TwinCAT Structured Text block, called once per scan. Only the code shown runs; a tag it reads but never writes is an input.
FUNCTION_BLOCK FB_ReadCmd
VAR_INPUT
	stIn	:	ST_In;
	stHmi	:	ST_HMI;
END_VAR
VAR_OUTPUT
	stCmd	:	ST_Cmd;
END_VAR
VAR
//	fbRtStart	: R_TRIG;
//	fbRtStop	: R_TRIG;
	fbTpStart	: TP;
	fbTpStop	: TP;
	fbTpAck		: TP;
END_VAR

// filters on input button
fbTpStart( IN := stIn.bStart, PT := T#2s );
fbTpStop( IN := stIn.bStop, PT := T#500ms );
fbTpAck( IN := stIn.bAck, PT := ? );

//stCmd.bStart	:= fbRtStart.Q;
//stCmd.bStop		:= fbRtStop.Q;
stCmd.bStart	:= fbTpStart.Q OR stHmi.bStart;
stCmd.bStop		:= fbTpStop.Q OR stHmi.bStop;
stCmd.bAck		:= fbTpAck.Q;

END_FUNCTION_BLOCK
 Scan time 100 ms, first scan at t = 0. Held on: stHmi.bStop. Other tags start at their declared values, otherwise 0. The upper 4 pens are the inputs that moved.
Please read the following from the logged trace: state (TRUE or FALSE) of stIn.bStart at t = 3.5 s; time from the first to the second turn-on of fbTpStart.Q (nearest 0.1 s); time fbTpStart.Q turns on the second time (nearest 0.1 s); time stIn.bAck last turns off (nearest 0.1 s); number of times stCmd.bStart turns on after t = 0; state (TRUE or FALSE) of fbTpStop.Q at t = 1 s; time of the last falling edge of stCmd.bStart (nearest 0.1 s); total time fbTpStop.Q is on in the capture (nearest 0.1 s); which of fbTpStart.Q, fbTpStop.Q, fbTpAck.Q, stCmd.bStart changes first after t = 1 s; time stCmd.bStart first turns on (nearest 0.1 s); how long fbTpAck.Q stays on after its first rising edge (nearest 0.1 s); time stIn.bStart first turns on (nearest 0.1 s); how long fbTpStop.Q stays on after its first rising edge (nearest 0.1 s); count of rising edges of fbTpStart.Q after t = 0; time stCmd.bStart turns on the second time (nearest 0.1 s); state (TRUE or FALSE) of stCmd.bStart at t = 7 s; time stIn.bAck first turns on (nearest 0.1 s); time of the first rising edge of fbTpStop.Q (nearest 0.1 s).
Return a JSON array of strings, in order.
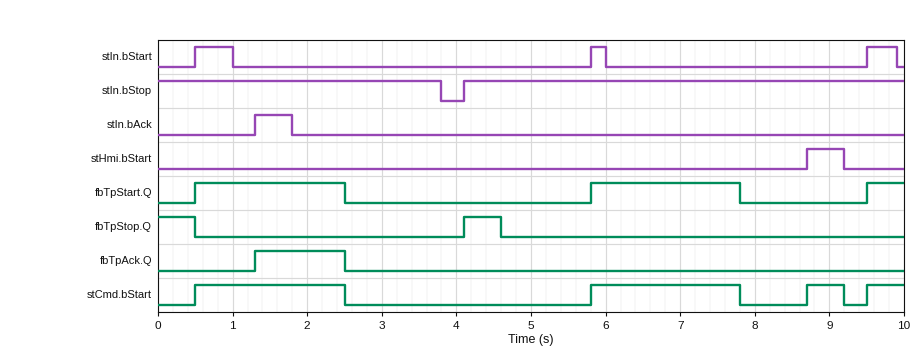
["FALSE", "5.3 s", "5.8 s", "1.8 s", "4", "FALSE", "9.2 s", "1.0 s", "fbTpAck.Q", "0.5 s", "1.2 s", "0.5 s", "0.5 s", "3", "5.8 s", "TRUE", "1.3 s", "4.1 s"]
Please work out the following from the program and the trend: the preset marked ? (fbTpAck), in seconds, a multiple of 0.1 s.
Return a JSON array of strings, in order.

["1.2 s"]
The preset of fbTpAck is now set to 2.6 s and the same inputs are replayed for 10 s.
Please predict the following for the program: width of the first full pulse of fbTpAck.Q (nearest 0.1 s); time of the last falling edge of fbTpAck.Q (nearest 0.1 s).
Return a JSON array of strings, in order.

["2.6 s", "3.9 s"]
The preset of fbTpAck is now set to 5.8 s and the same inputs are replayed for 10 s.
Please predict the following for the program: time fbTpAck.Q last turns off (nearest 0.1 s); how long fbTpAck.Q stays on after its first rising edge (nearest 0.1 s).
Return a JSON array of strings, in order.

["7.1 s", "5.8 s"]
